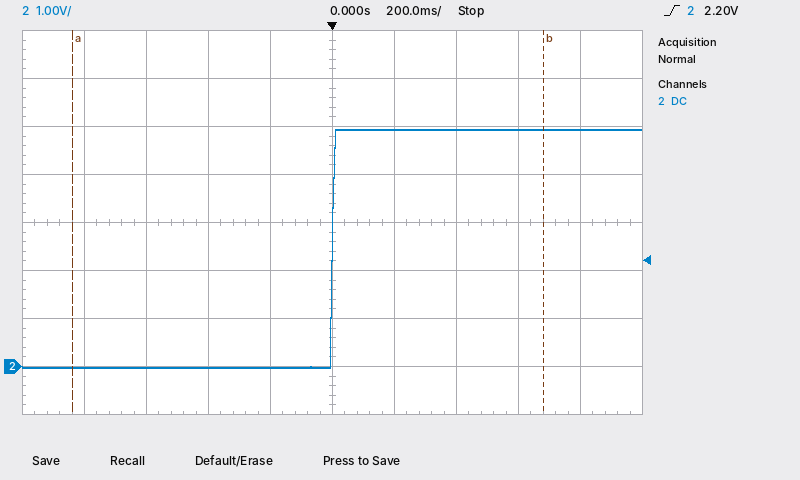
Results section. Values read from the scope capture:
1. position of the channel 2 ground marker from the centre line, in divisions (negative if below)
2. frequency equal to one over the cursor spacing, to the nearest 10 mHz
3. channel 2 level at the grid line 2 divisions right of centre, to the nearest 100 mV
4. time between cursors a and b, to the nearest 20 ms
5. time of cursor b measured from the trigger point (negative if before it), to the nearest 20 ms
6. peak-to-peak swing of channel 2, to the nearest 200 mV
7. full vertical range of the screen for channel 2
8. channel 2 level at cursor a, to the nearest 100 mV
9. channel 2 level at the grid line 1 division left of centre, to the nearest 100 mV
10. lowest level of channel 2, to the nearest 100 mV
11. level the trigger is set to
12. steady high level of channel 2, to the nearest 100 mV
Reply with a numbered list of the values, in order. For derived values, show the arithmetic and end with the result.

1. -3.0 div
2. 1 / 1.52 s ≈ 660 mHz
3. 4.9 V
4. 1.52 s
5. +680 ms
6. 5.0 V
7. 8 V
8. 0.0 V
9. 0.0 V
10. 0.0 V
11. 2.20 V
12. 4.9 V
